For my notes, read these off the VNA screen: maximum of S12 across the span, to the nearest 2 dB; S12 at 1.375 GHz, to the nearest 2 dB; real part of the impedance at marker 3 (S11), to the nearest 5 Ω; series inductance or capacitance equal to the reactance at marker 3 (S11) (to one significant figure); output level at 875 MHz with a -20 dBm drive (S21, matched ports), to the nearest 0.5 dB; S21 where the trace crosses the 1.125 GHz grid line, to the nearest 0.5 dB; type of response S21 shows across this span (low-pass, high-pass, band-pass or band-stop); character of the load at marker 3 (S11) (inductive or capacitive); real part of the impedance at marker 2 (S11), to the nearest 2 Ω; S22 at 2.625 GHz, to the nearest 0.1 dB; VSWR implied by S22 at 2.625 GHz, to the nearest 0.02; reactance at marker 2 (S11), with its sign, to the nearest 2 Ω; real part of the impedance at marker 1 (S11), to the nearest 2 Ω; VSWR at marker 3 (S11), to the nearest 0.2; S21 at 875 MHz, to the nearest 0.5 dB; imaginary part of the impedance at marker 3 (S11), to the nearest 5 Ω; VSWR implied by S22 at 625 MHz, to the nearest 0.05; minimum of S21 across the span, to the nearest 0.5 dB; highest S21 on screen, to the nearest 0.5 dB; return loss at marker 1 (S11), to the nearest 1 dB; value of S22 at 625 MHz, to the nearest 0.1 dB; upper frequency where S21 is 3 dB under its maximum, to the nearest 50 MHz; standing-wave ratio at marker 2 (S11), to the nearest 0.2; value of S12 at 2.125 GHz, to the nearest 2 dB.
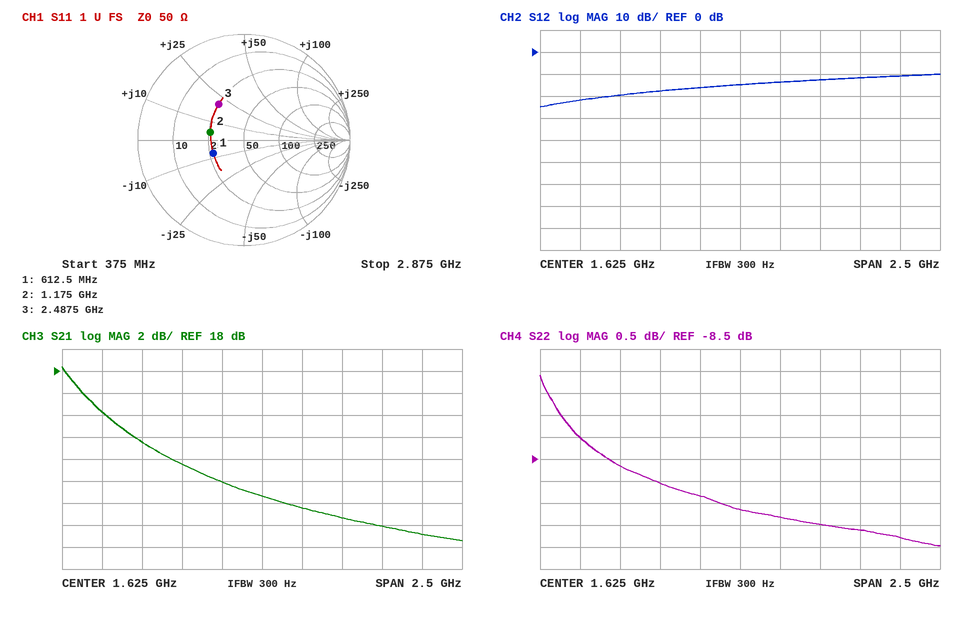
-10 dB
-16 dB
25 Ω
1 nH
-8.5 dBm
9.5 dB
low-pass
inductive
26 Ω
-10.3 dB
1.88
+4 Ω
26 Ω
2.4
11.5 dB
+20 Ω
2.30
2.5 dB
18.5 dB
10 dB
-8.0 dB
550 MHz
2.0
-12 dB
